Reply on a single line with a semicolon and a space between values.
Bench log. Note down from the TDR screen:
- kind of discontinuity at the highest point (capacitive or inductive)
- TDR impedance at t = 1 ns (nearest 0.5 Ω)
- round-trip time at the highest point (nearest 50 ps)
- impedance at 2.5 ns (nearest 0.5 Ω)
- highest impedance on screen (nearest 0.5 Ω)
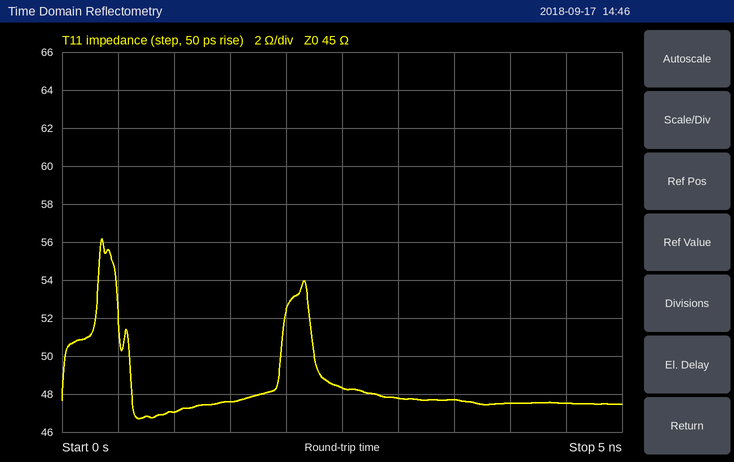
inductive; 47.0 Ω; 350 ps; 48.5 Ω; 56.0 Ω
